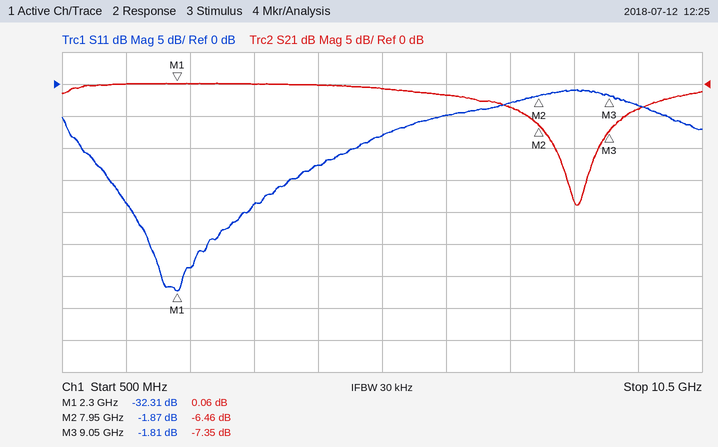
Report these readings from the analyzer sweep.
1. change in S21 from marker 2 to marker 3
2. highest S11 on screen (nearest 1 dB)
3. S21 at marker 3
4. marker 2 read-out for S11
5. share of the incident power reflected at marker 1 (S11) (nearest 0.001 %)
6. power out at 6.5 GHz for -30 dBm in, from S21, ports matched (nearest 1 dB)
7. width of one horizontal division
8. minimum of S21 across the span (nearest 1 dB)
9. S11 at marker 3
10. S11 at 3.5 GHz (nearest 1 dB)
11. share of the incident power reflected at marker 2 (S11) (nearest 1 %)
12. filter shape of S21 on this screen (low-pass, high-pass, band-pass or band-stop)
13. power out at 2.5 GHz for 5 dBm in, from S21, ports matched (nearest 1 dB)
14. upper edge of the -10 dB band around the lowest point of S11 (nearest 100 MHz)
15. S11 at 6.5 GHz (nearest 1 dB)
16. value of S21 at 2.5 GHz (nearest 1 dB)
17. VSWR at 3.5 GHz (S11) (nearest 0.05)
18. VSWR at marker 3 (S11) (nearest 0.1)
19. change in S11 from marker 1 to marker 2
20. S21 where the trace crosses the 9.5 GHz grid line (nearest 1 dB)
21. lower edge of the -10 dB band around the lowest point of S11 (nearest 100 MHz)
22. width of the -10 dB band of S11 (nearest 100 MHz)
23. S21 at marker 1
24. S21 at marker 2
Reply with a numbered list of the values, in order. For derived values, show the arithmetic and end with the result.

1. -7.35 − (-6.46) = -0.89 dB
2. -1 dB
3. -7.35 dB
4. -1.87 dB
5. 10^(-32.31/10) ≈ 0.059 %
6. -30 dBm + (-2 dB) = -32 dBm
7. 1 GHz
8. -19 dB
9. -1.81 dB
10. -19 dB
11. 10^(-1.87/10) ≈ 65 %
12. band-stop
13. 5 dBm + (0 dB) = 5 dBm
14. 5.1 GHz
15. -5 dB
16. 0 dB
17. |Γ| = 10^(-19/20) = 0.1122; VSWR = (1 + 0.1122)/(1 − 0.1122) ≈ 1.25
18. (1 + 0.8119)/(1 − 0.8119) ≈ 9.6
19. -1.87 − (-32.31) = 30.44 dB
20. -4 dB
21. 800 MHz
22. 5.1 GHz − 800 MHz = 4.3 GHz
23. 0.06 dB
24. -6.46 dB
